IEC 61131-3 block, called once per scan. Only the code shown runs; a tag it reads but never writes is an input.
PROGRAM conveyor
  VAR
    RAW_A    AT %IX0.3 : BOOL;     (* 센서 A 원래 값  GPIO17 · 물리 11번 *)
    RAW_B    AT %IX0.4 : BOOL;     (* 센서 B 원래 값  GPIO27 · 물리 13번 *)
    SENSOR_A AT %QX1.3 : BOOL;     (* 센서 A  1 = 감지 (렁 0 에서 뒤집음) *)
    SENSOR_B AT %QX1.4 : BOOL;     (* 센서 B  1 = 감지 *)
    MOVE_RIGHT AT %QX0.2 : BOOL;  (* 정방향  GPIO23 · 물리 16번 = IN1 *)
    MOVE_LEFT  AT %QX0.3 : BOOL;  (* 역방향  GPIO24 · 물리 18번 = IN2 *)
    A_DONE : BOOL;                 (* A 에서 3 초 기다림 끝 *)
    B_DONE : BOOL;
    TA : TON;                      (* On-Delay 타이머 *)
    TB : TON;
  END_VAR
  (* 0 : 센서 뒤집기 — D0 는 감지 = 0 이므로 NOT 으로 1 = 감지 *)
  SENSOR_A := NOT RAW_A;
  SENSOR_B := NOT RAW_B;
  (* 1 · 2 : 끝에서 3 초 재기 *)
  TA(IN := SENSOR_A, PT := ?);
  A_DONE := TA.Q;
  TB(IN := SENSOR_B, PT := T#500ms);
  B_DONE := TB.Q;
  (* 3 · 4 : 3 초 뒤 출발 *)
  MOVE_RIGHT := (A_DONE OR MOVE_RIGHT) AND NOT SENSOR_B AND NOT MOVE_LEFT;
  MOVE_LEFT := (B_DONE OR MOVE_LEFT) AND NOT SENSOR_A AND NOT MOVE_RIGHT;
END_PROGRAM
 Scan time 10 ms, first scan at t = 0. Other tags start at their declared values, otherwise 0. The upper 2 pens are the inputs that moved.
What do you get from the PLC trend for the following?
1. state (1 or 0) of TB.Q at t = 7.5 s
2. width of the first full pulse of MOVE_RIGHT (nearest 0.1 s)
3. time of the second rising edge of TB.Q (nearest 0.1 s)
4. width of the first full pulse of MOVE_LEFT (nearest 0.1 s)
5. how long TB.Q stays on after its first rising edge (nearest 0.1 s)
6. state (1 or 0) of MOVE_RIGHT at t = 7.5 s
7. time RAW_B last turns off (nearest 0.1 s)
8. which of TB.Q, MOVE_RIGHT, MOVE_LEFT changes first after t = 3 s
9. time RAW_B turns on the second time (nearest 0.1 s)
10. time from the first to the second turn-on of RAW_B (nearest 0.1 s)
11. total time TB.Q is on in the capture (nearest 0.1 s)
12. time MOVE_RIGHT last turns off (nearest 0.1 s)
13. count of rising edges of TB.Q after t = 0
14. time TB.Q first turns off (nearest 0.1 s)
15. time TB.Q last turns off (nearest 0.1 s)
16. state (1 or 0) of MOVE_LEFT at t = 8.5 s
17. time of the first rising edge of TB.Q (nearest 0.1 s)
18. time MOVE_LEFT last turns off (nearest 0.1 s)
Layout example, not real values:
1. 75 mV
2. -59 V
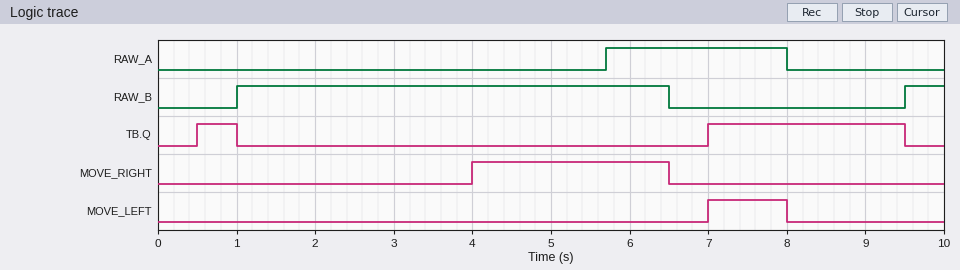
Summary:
1. 1
2. 2.5 s
3. 7.0 s
4. 1.0 s
5. 0.5 s
6. 0
7. 6.5 s
8. MOVE_RIGHT
9. 9.5 s
10. 8.5 s
11. 3.0 s
12. 6.5 s
13. 2
14. 1.0 s
15. 9.5 s
16. 0
17. 0.5 s
18. 8.0 s
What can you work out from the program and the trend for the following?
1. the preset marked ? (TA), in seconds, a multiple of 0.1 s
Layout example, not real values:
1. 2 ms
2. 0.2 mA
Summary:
1. 4.0 s
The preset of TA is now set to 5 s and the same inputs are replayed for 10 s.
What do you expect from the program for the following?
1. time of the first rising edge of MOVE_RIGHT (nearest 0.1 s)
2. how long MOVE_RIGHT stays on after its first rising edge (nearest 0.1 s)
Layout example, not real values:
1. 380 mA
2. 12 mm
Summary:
1. 5.0 s
2. 1.5 s
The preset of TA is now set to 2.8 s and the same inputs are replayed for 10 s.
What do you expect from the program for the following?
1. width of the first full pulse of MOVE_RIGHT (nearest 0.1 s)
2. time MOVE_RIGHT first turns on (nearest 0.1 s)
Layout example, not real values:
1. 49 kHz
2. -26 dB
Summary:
1. 3.7 s
2. 2.8 s
